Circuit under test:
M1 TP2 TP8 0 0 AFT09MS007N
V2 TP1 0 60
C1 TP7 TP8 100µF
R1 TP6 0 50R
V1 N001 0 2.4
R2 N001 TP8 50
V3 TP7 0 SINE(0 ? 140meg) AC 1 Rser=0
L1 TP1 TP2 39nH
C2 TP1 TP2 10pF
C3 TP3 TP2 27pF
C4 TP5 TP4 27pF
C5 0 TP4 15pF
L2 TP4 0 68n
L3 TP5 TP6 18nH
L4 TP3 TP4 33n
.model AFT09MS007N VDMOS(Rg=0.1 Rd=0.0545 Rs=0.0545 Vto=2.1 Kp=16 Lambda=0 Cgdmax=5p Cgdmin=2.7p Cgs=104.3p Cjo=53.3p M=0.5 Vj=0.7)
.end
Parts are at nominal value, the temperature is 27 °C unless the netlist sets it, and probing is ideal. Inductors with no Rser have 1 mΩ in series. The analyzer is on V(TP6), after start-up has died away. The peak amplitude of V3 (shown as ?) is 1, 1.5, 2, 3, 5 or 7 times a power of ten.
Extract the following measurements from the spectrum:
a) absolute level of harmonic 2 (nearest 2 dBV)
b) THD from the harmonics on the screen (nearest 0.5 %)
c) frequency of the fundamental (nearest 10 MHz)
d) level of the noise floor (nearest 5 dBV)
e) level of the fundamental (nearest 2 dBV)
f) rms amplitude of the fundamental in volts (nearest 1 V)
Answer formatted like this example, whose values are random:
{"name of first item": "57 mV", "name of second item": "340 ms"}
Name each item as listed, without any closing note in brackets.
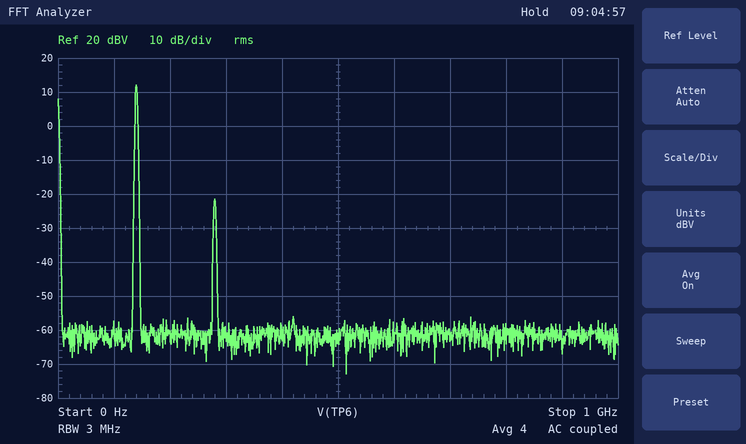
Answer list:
{"absolute level of harmonic 2": "-22 dBV", "THD from the harmonics on the screen": "2.0 %", "frequency of the fundamental": "140 MHz", "level of the noise floor": "-60 dBV", "level of the fundamental": "12 dBV", "rms amplitude of the fundamental in volts": "4 V"}
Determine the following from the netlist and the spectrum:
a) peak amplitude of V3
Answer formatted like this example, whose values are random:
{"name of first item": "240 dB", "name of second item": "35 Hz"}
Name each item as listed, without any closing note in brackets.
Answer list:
{"peak amplitude of V3": "30 mV"}
